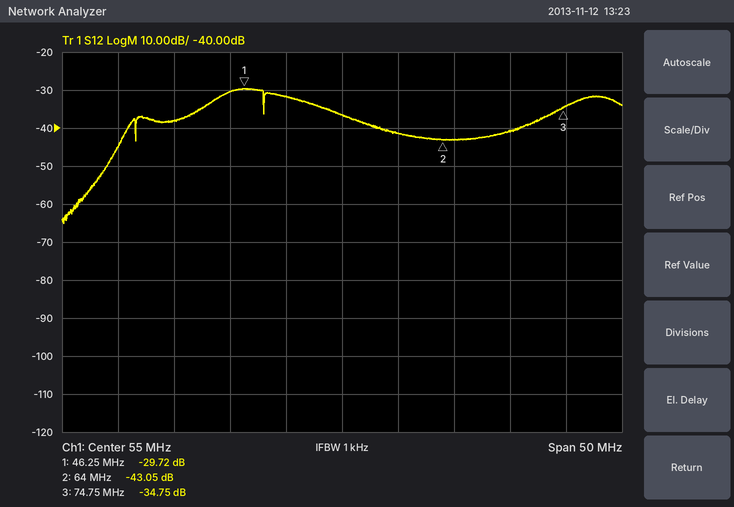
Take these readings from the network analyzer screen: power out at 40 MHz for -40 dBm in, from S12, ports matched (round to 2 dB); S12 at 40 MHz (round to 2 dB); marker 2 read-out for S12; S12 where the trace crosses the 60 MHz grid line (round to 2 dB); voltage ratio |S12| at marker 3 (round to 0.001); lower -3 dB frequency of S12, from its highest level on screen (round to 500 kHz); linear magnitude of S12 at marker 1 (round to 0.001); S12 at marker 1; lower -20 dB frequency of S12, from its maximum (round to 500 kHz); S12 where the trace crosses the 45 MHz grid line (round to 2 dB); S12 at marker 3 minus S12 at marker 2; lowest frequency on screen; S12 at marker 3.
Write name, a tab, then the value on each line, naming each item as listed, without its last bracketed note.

power out at 40 MHz for -40 dBm in, from S12, ports matched	-78 dBm
S12 at 40 MHz	-38 dB
marker 2 read-out for S12	-43.05 dB
S12 where the trace crosses the 60 MHz grid line	-42 dB
voltage ratio |S12| at marker 3	0.018
lower -3 dB frequency of S12, from its highest level on screen	43.5 MHz
linear magnitude of S12 at marker 1	0.033
S12 at marker 1	-29.72 dB
lower -20 dB frequency of S12, from its maximum	34.0 MHz
S12 where the trace crosses the 45 MHz grid line	-30 dB
S12 at marker 3 minus S12 at marker 2	8.30 dB
lowest frequency on screen	30 MHz
S12 at marker 3	-34.75 dB
